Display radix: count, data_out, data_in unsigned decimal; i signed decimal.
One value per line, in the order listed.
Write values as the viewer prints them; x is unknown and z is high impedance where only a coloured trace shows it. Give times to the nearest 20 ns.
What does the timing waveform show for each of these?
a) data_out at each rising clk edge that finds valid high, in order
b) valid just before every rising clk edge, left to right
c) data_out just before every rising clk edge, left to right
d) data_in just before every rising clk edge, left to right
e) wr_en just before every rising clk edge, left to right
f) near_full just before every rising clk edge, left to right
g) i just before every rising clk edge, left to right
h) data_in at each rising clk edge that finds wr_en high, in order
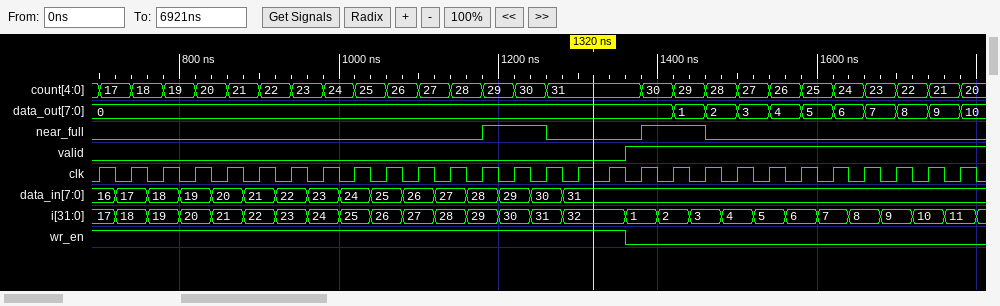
0, 0, 1, 2, 3, 4, 5, 6, 7, 8, 9
0 0 0 0 0 0 0 0 0 0 0 0 0 0 0 0 0 1 1 1 1 1 1 1 1 1 1 1
0, 0, 0, 0, 0, 0, 0, 0, 0, 0, 0, 0, 0, 0, 0, 0, 0, 0, 0, 1, 2, 3, 4, 5, 6, 7, 8, 9
16, 17, 18, 19, 20, 21, 22, 23, 24, 25, 26, 27, 28, 29, 30, 31, 31, 31, 31, 31, 31, 31, 31, 31, 31, 31, 31, 31
1 1 1 1 1 1 1 1 1 1 1 1 1 1 1 1 1 0 0 0 0 0 0 0 0 0 0 0
0 0 0 0 0 0 0 0 0 0 0 0 0 1 1 0 0 0 1 1 0 0 0 0 0 0 0 0
17, 18, 19, 20, 21, 22, 23, 24, 25, 26, 27, 28, 29, 30, 31, 32, 32, 1, 2, 3, 4, 5, 6, 7, 8, 9, 10, 11
16, 17, 18, 19, 20, 21, 22, 23, 24, 25, 26, 27, 28, 29, 30, 31, 31
